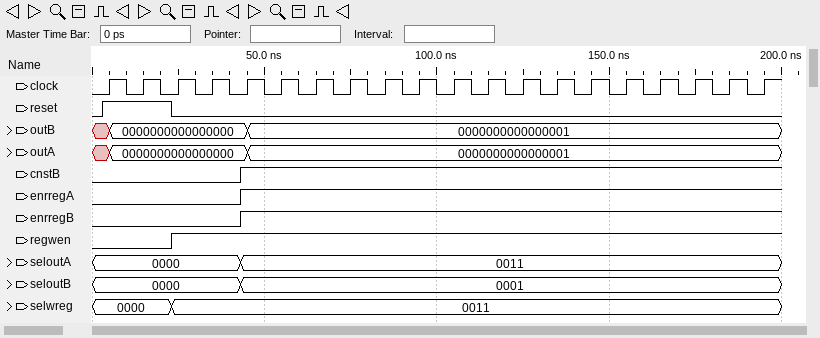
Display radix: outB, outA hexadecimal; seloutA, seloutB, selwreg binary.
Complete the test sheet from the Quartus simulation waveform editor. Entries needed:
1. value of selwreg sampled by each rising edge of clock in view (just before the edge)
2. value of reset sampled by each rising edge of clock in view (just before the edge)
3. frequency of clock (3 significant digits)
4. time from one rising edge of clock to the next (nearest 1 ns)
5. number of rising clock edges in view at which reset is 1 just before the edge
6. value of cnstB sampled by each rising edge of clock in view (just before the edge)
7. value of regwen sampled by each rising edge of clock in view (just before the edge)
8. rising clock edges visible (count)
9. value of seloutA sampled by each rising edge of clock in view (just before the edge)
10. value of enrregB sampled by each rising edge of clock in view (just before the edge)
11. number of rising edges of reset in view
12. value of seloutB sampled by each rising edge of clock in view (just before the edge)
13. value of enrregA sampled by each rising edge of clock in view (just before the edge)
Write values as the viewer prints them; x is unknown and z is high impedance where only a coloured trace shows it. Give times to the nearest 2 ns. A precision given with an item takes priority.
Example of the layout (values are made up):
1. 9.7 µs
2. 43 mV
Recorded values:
1. 0000, 0000, 0011, 0011, 0011, 0011, 0011, 0011, 0011, 0011, 0011, 0011, 0011, 0011, 0011, 0011, 0011, 0011, 0011, 0011
2. 1 1 0 0 0 0 0 0 0 0 0 0 0 0 0 0 0 0 0 0
3. 100 MHz
4. 10 ns
5. 2
6. 0 0 0 0 1 1 1 1 1 1 1 1 1 1 1 1 1 1 1 1
7. 0 0 1 1 1 1 1 1 1 1 1 1 1 1 1 1 1 1 1 1
8. 20
9. 0000, 0000, 0000, 0000, 0011, 0011, 0011, 0011, 0011, 0011, 0011, 0011, 0011, 0011, 0011, 0011, 0011, 0011, 0011, 0011
10. 0 0 0 0 1 1 1 1 1 1 1 1 1 1 1 1 1 1 1 1
11. 1
12. 0000, 0000, 0000, 0000, 0001, 0001, 0001, 0001, 0001, 0001, 0001, 0001, 0001, 0001, 0001, 0001, 0001, 0001, 0001, 0001
13. 0 0 0 0 1 1 1 1 1 1 1 1 1 1 1 1 1 1 1 1
